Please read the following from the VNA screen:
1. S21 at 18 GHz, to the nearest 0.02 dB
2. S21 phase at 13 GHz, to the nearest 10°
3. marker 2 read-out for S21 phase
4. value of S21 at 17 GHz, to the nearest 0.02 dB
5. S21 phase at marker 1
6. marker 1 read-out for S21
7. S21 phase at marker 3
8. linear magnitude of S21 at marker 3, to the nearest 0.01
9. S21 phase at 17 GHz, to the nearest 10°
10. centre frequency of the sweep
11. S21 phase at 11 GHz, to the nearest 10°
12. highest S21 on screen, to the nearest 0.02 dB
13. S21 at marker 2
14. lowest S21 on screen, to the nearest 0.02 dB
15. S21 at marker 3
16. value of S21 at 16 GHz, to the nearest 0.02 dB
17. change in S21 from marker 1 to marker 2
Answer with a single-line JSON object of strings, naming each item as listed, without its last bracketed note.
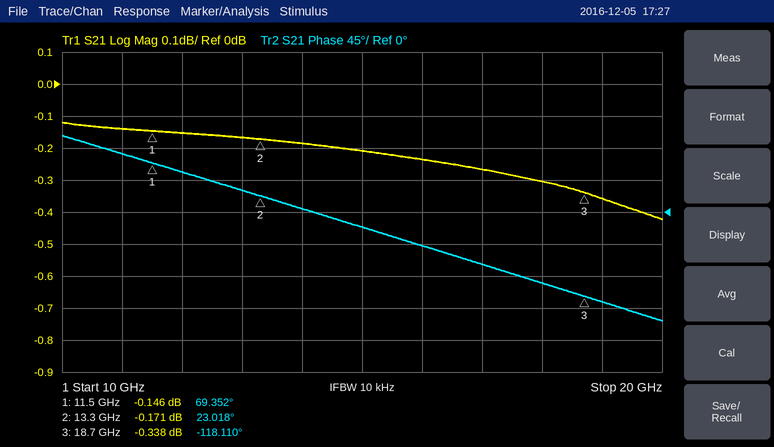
{"S21 at 18 GHz, to the nearest 0.02 dB": "-0.30 dB", "S21 phase at 13 GHz, to the nearest 10°": "30°", "marker 2 read-out for S21 phase": "23.018°", "value of S21 at 17 GHz, to the nearest 0.02 dB": "-0.26 dB", "S21 phase at marker 1": "69.352°", "marker 1 read-out for S21": "-0.146 dB", "S21 phase at marker 3": "-118.110°", "linear magnitude of S21 at marker 3, to the nearest 0.01": "0.96", "S21 phase at 17 GHz, to the nearest 10°": "-70°", "centre frequency of the sweep": "15 GHz", "S21 phase at 11 GHz, to the nearest 10°": "80°", "highest S21 on screen, to the nearest 0.02 dB": "-0.12 dB", "S21 at marker 2": "-0.171 dB", "lowest S21 on screen, to the nearest 0.02 dB": "-0.42 dB", "S21 at marker 3": "-0.338 dB", "value of S21 at 16 GHz, to the nearest 0.02 dB": "-0.24 dB", "change in S21 from marker 1 to marker 2": "-0.025 dB"}
